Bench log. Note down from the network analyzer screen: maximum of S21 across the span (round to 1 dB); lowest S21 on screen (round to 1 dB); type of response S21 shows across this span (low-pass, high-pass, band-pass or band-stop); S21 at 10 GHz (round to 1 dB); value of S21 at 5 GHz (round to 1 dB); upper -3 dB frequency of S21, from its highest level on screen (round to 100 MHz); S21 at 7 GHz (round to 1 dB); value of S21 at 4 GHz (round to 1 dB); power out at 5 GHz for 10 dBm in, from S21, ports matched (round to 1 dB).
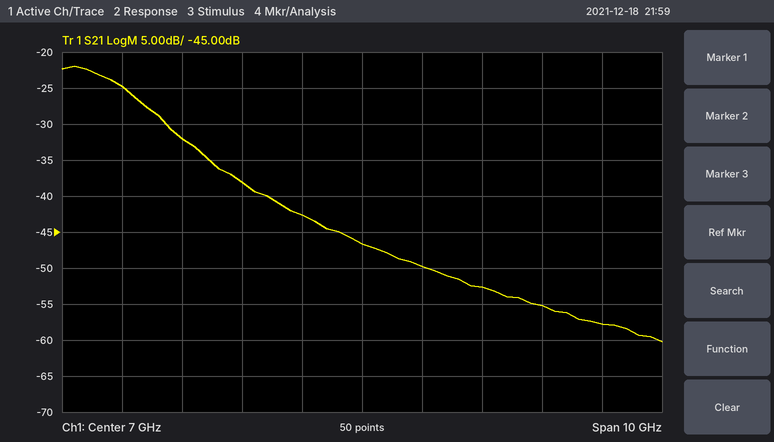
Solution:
-22 dB
-60 dB
low-pass
-55 dB
-38 dB
3.0 GHz
-47 dB
-32 dB
-28 dBm
